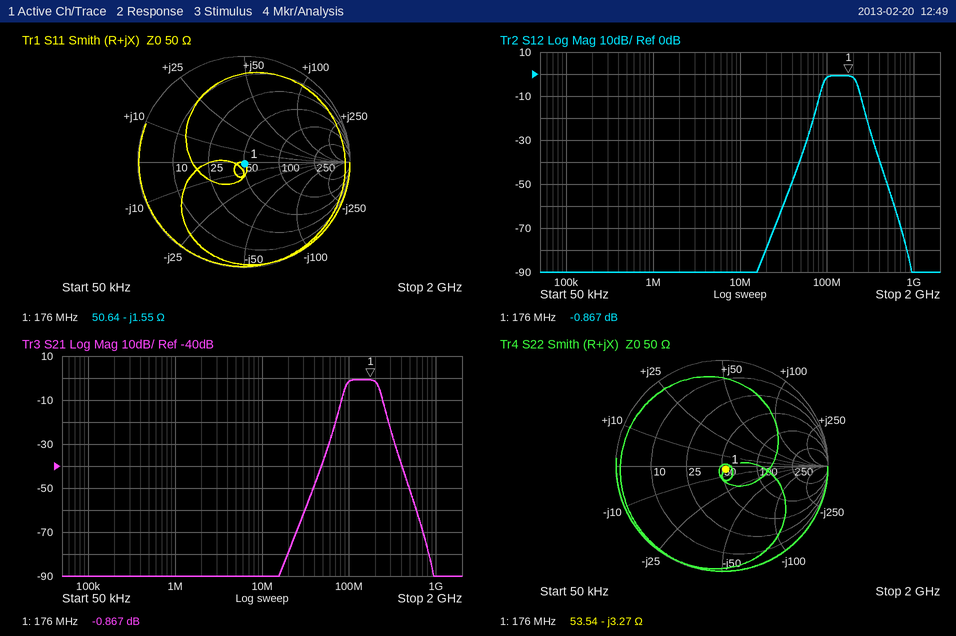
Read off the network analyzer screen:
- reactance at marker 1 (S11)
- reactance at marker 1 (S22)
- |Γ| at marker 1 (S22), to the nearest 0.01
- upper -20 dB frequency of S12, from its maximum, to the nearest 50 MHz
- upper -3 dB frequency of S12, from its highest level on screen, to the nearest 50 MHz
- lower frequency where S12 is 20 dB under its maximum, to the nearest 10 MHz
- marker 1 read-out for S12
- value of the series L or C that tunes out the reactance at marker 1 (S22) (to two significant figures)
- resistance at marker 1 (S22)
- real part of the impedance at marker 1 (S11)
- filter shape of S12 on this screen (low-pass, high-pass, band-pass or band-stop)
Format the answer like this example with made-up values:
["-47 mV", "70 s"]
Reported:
["-1.55 Ω", "-3.27 Ω", "0.05", "300 MHz", "200 MHz", "70 MHz", "-0.867 dB", "3.0 nH", "53.54 Ω", "50.64 Ω", "band-pass"]
